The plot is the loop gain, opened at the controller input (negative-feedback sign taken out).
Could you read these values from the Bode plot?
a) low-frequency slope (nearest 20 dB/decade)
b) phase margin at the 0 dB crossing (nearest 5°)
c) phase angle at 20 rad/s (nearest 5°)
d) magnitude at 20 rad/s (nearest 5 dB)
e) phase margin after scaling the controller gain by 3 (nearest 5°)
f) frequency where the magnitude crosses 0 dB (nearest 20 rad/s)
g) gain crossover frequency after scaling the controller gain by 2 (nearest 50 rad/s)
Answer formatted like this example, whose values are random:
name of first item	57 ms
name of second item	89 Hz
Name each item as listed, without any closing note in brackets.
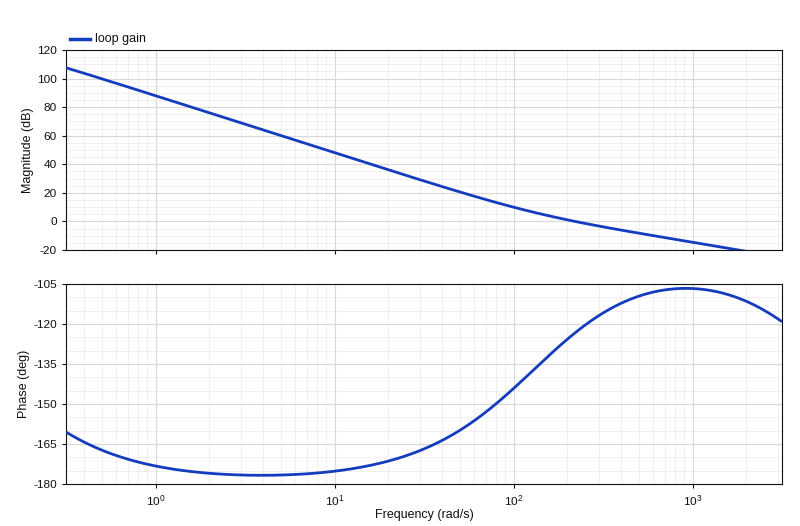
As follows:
low-frequency slope	-40 dB/decade
phase margin at the 0 dB crossing	55°
phase angle at 20 rad/s	-170°
magnitude at 20 rad/s	35 dB
phase margin after scaling the controller gain by 3	70°
frequency where the magnitude crosses 0 dB	220 rad/s
gain crossover frequency after scaling the controller gain by 2	400 rad/s
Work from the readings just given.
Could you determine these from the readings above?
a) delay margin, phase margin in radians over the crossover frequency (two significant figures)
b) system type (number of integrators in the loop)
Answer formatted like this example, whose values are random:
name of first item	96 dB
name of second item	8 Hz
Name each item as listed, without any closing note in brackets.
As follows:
delay margin, phase margin in radians over the crossover frequency	0.0044 s
system type	2
